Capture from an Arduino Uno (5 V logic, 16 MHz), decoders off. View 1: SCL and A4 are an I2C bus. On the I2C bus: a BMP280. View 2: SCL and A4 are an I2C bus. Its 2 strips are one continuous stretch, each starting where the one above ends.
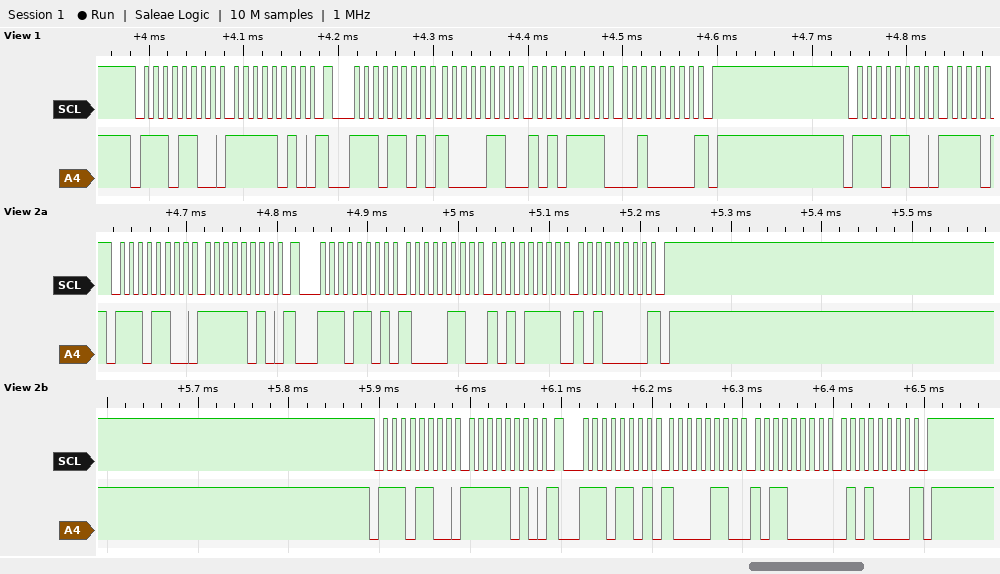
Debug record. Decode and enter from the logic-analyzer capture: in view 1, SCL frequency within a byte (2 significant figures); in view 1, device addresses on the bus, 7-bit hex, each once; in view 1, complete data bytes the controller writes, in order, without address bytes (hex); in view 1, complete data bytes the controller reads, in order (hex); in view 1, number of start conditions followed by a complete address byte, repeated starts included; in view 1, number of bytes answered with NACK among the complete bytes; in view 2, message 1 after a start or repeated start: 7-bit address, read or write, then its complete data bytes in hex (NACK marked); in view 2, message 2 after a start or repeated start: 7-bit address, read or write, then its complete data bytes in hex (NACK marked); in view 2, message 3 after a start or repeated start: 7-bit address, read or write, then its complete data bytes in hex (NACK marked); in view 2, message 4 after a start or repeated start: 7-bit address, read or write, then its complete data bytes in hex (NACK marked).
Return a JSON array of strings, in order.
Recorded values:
["100 kHz", "0x76", "FA", "86 AF 20", "3", "1", "0x76 write: FA", "0x76 read: 86 AF A0 NACK", "0x76 write: FA", "0x76 read: 86 B0 50 NACK"]
